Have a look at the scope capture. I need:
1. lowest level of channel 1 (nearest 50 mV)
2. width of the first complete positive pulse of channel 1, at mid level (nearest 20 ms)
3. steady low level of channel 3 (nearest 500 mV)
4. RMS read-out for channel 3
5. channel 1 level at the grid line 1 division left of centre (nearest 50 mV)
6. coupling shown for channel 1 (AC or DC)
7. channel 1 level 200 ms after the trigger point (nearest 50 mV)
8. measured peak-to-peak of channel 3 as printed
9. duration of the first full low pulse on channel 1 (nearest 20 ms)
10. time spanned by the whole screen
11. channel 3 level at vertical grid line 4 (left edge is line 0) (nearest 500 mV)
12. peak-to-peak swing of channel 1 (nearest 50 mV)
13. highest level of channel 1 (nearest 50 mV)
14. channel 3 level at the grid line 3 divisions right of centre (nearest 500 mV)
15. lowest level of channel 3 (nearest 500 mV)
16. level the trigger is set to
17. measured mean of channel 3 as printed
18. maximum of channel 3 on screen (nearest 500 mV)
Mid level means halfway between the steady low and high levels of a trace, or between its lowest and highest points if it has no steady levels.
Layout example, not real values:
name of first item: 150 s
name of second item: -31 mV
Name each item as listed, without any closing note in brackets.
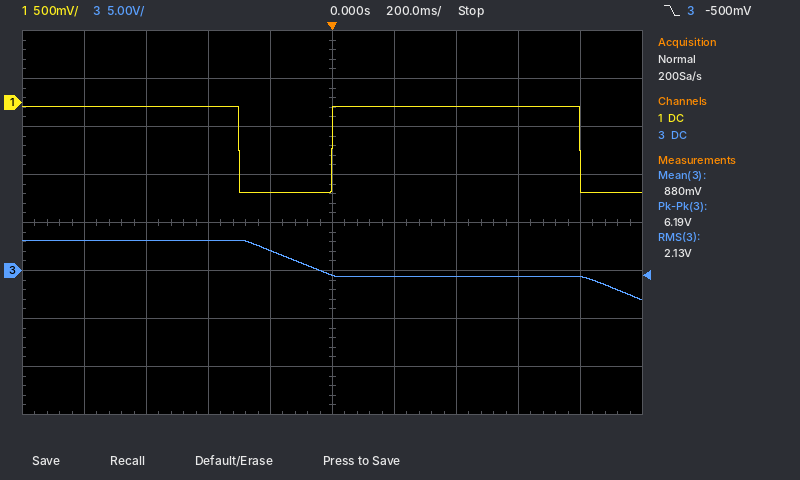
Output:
lowest level of channel 1: -950 mV
width of the first complete positive pulse of channel 1, at mid level: 800 ms
steady low level of channel 3: -500 mV
RMS read-out for channel 3: 2.13 V
channel 1 level at the grid line 1 division left of centre: -950 mV
coupling shown for channel 1: DC
channel 1 level 200 ms after the trigger point: -50 mV
measured peak-to-peak of channel 3 as printed: 6.19 V
duration of the first full low pulse on channel 1: 300 ms
time spanned by the whole screen: 2 s
channel 3 level at vertical grid line 4 (left edge is line 0): 2.0 V
peak-to-peak swing of channel 1: 900 mV
highest level of channel 1: -50 mV
channel 3 level at the grid line 3 divisions right of centre: -500 mV
lowest level of channel 3: -3.0 V
level the trigger is set to: -500 mV
measured mean of channel 3 as printed: 880 mV
maximum of channel 3 on screen: 3.0 V
